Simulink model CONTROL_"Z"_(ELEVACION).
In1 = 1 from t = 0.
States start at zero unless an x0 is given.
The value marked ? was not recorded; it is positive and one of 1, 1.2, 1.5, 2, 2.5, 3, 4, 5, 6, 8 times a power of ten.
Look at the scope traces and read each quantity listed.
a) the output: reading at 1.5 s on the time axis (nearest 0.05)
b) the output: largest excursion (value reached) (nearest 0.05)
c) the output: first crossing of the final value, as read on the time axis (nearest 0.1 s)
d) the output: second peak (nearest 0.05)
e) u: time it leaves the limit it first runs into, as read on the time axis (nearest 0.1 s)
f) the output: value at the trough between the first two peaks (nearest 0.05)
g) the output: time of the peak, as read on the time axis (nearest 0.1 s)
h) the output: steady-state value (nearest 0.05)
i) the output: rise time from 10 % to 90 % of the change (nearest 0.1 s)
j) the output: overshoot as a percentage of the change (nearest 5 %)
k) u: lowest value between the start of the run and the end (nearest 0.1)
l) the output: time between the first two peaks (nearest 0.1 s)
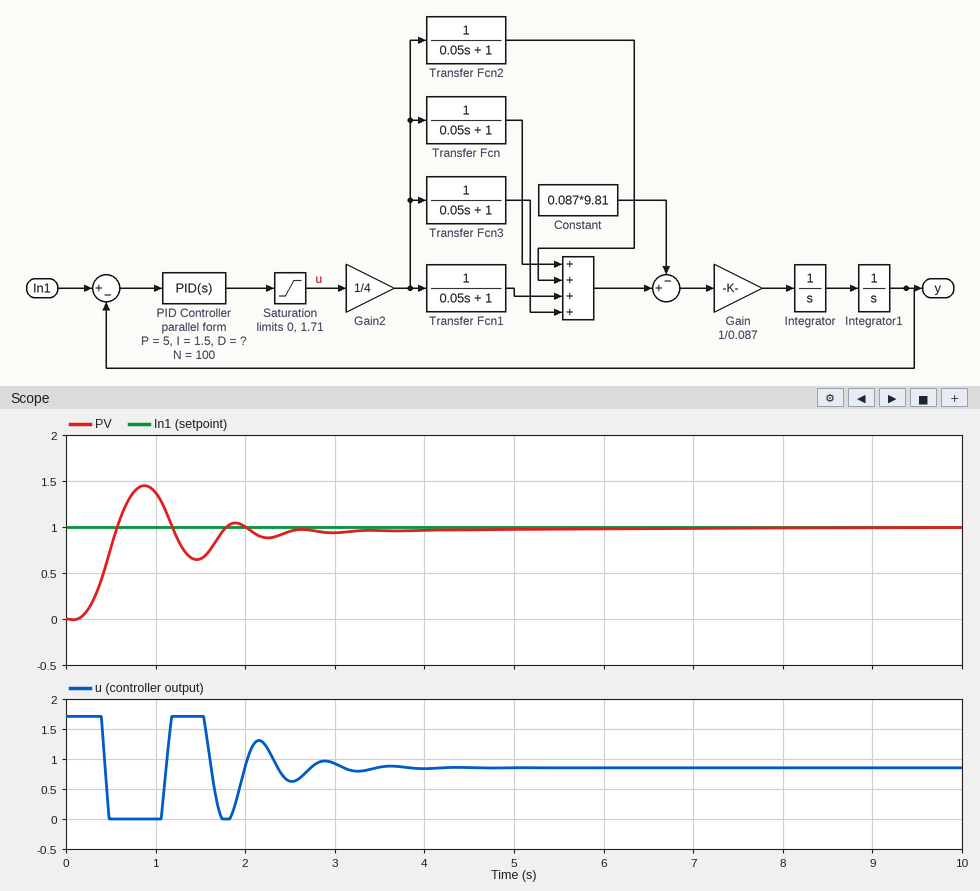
0.65
1.45
0.6 s
1.05
0.4 s
0.65
0.9 s
1.00
0.3 s
45 %
0.0
1.0 s
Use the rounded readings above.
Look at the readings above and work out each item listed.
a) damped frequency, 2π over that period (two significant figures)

6.3 rad/s
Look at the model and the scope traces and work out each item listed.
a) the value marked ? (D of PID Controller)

0.6
